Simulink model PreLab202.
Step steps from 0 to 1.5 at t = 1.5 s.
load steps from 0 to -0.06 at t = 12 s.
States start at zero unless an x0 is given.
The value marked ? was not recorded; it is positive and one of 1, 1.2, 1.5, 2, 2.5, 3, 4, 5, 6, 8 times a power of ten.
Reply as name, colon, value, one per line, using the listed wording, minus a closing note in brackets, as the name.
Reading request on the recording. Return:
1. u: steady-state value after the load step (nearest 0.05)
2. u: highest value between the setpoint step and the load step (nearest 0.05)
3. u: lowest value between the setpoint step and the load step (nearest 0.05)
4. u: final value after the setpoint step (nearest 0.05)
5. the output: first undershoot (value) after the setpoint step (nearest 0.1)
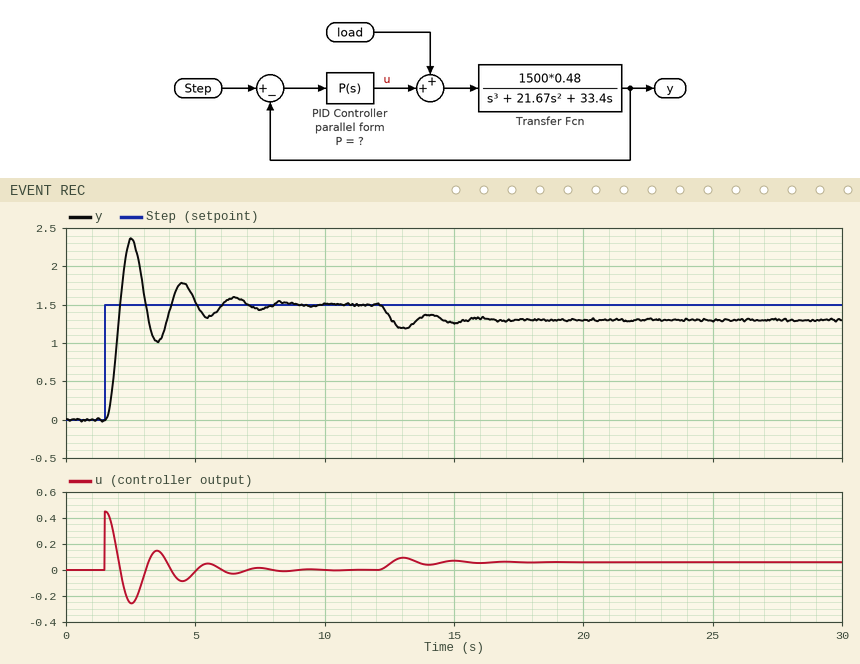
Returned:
u: steady-state value after the load step: 0.05
u: highest value between the setpoint step and the load step: 0.45
u: lowest value between the setpoint step and the load step: -0.25
u: final value after the setpoint step: 0.00
the output: first undershoot (value) after the setpoint step: 1.0
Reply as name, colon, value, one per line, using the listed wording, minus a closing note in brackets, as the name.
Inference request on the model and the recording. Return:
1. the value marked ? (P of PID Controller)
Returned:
the value marked ?: 0.3
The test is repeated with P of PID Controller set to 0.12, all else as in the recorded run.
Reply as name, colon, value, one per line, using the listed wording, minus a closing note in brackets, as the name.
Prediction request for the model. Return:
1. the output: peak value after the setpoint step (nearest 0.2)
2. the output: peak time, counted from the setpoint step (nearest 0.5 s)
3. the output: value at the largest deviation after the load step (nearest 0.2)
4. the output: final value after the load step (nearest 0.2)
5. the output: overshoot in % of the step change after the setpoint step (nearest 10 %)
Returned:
the output: peak value after the setpoint step: 2.0
the output: peak time, counted from the setpoint step: 1.5 s
the output: value at the largest deviation after the load step: 0.8
the output: final value after the load step: 1.0
the output: overshoot in % of the step change after the setpoint step: 30 %
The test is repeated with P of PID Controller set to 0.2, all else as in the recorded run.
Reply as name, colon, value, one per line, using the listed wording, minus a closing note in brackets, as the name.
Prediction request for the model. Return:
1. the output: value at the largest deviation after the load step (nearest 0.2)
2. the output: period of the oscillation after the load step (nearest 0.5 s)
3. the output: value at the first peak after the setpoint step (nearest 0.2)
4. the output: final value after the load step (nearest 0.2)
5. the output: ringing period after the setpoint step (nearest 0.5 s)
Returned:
the output: value at the largest deviation after the load step: 1.0
the output: period of the oscillation after the load step: 2.5 s
the output: value at the first peak after the setpoint step: 2.2
the output: final value after the load step: 1.2
the output: ringing period after the setpoint step: 2.5 s
